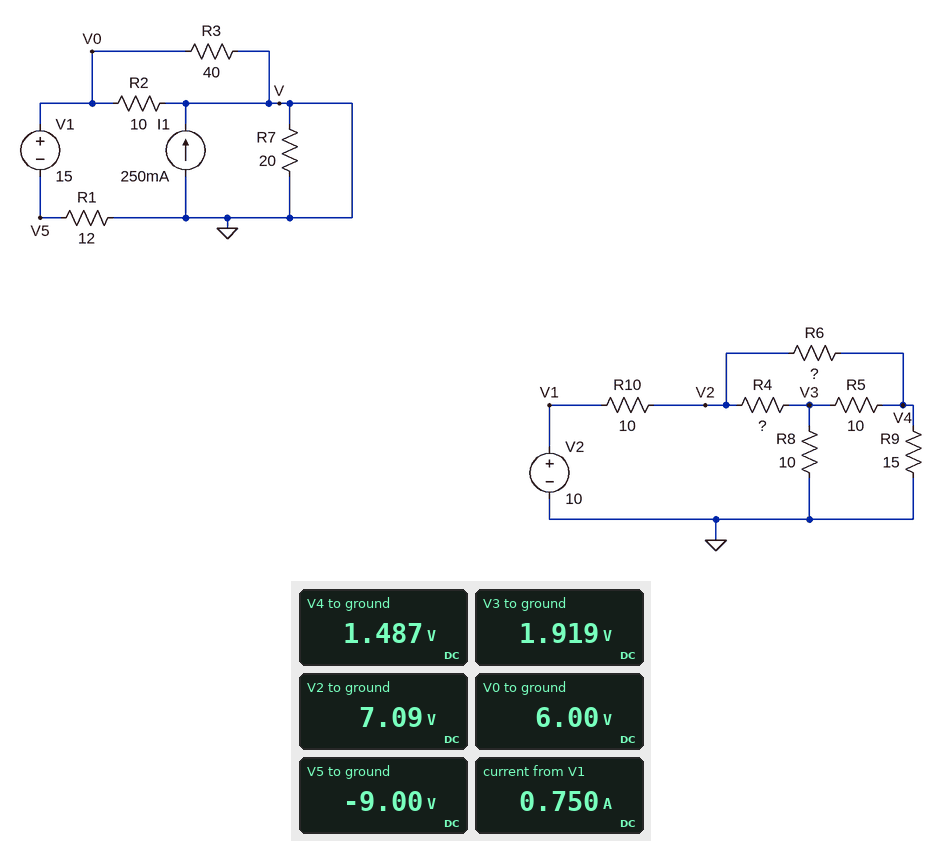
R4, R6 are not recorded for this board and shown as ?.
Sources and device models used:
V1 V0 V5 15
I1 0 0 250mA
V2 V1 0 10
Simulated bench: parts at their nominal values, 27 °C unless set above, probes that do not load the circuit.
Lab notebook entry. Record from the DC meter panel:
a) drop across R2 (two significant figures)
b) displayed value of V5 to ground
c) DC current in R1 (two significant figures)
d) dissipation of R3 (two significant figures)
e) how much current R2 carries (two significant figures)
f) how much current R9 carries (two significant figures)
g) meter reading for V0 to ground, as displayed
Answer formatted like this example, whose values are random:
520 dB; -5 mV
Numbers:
6.0 V; -9.00 V; 750 mA; 900 mW; 600 mA; 99 mA; 6.00 V
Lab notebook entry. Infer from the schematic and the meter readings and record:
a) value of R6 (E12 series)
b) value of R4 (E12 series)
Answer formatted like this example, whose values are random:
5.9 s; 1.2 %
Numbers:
100 Ω; 22 Ω
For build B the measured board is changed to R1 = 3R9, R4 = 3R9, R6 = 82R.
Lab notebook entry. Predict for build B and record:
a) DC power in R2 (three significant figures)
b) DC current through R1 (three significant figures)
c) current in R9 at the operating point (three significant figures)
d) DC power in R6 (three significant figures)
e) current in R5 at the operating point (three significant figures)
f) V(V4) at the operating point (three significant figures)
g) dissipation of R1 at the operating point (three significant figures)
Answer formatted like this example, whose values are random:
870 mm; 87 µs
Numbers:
10.2 W; 1.26 A; 149 mA; 102 mW; 114 mA; 2.24 V; 6.20 W
